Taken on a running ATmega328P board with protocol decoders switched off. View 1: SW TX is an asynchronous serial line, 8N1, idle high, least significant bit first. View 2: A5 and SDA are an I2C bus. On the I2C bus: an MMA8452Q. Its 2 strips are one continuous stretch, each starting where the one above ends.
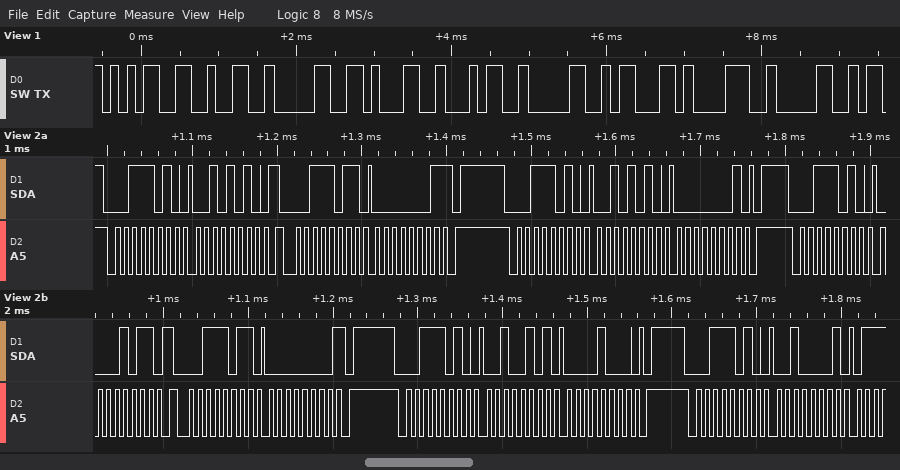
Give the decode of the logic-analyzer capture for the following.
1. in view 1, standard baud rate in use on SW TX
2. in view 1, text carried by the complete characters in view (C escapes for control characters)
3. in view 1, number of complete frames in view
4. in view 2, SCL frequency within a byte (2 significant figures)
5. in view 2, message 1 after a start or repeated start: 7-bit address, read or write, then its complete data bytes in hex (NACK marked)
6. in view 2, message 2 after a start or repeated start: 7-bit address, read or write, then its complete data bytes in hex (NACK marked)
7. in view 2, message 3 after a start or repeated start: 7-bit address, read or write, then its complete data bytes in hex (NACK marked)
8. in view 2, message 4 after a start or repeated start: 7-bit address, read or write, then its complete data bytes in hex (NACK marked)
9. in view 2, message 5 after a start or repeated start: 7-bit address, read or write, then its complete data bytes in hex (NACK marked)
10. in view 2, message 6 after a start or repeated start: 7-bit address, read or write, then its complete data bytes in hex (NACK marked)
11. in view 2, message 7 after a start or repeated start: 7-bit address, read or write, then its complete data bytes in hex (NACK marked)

9600 baud
"520140c80"
9
100 kHz
0x1D write: 2A
0x1D read: 01 NACK
0x1D write: 2A 01
0x1D write: 0B
0x1D read: 00 NACK
0x1D write: 25 08
0x1D write: 21
